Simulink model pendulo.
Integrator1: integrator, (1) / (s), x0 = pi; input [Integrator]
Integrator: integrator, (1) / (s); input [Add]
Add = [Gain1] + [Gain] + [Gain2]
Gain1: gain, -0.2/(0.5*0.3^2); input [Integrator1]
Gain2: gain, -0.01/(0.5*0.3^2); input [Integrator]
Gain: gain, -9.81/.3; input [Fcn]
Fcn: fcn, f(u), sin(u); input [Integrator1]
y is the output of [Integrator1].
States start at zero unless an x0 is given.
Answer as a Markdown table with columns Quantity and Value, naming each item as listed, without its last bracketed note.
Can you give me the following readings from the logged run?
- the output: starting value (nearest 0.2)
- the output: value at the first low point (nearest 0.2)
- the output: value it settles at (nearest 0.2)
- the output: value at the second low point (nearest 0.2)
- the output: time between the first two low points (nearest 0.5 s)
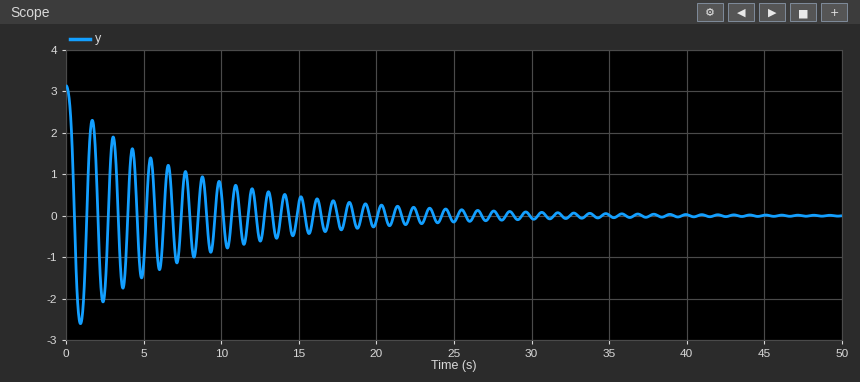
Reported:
| Quantity | Value |
|---|---|
| the output: starting value | 3.2 |
| the output: value at the first low point | -2.6 |
| the output: value it settles at | 0.0 |
| the output: value at the second low point | -2.0 |
| the output: time between the first two low points | 1.5 s |
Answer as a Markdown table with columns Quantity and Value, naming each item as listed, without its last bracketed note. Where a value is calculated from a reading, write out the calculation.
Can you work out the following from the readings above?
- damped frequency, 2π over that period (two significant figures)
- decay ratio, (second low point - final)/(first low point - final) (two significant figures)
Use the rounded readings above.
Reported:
| Quantity | Value |
|---|---|
| damped frequency, 2π over that period | 2π / 1.5 = 4.2 rad/s |
| decay ratio, (second low point - final)/(first low point - final) | (-2 - 0) / (-2.6 - 0) = 0.77 |
